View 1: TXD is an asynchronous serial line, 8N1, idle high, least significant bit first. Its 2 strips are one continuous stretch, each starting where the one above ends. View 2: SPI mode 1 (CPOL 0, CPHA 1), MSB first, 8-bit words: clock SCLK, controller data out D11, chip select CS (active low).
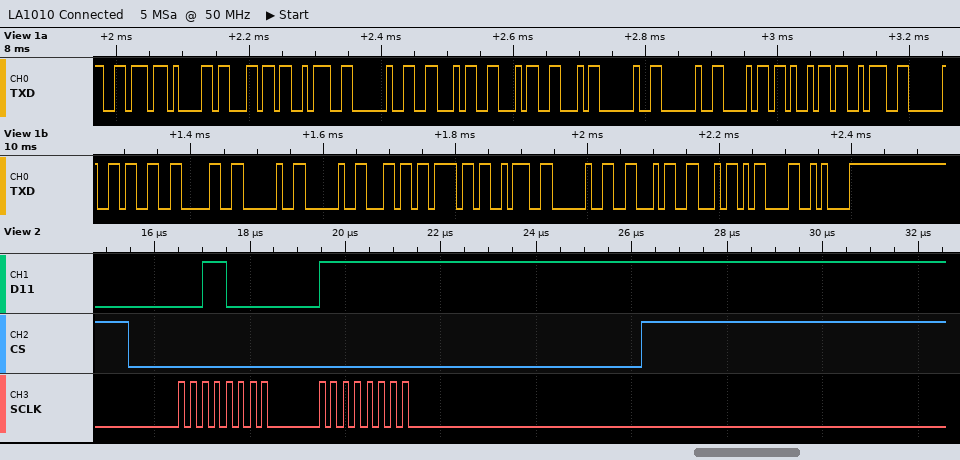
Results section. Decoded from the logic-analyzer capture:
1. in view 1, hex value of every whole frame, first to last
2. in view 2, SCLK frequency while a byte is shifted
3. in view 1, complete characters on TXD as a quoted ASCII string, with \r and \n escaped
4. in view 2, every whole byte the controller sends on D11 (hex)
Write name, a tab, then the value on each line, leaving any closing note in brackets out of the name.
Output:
in view 1, hex value of every whole frame, first to last	76 61 6C 3A 20 46 46 46 20 20 68 69 3A 20 33 30 20 20 6C 6F 3A 20 46 46 0D 0A
in view 2, SCLK frequency while a byte is shifted	4 MHz
in view 1, complete characters on TXD as a quoted ASCII string, with \r and \n escaped	"val: FFF  hi: 30  lo: FF\r\n"
in view 2, every whole byte the controller sends on D11	30 FF
